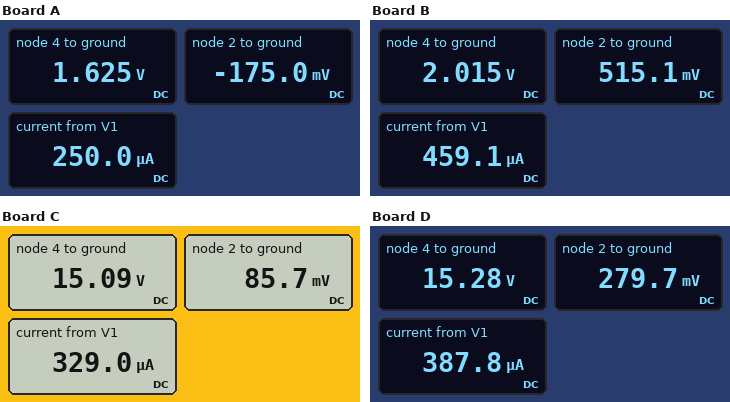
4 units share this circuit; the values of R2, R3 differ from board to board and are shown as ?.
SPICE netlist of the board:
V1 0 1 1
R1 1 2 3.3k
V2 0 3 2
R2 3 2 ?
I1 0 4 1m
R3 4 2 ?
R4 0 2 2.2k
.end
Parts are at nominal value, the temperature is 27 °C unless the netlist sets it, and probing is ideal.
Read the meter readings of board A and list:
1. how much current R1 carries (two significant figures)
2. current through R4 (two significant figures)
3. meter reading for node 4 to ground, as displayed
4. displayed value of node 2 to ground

250 µA
80 µA
1.625 V
-175.0 mV
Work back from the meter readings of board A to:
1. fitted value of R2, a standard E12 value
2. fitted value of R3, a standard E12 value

2.2 kΩ
1.8 kΩ
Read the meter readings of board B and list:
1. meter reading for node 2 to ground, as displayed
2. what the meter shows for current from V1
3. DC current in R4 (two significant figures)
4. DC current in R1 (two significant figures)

515.1 mV
459.1 µA
230 µA
460 µA
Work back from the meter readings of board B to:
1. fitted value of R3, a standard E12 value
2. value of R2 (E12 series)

1.5 kΩ
8.2 kΩ
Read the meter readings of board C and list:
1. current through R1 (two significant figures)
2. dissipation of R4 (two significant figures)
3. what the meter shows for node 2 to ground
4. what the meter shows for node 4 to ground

330 µA
3.3 µW
85.7 mV
15.09 V
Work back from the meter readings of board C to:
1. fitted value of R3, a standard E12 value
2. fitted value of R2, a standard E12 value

15 kΩ
3.3 kΩ
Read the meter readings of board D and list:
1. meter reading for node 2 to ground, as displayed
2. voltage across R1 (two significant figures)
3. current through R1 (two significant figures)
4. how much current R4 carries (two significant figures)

279.7 mV
1.3 V
390 µA
130 µA
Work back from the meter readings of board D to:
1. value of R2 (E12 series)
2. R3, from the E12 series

4.7 kΩ
15 kΩ
